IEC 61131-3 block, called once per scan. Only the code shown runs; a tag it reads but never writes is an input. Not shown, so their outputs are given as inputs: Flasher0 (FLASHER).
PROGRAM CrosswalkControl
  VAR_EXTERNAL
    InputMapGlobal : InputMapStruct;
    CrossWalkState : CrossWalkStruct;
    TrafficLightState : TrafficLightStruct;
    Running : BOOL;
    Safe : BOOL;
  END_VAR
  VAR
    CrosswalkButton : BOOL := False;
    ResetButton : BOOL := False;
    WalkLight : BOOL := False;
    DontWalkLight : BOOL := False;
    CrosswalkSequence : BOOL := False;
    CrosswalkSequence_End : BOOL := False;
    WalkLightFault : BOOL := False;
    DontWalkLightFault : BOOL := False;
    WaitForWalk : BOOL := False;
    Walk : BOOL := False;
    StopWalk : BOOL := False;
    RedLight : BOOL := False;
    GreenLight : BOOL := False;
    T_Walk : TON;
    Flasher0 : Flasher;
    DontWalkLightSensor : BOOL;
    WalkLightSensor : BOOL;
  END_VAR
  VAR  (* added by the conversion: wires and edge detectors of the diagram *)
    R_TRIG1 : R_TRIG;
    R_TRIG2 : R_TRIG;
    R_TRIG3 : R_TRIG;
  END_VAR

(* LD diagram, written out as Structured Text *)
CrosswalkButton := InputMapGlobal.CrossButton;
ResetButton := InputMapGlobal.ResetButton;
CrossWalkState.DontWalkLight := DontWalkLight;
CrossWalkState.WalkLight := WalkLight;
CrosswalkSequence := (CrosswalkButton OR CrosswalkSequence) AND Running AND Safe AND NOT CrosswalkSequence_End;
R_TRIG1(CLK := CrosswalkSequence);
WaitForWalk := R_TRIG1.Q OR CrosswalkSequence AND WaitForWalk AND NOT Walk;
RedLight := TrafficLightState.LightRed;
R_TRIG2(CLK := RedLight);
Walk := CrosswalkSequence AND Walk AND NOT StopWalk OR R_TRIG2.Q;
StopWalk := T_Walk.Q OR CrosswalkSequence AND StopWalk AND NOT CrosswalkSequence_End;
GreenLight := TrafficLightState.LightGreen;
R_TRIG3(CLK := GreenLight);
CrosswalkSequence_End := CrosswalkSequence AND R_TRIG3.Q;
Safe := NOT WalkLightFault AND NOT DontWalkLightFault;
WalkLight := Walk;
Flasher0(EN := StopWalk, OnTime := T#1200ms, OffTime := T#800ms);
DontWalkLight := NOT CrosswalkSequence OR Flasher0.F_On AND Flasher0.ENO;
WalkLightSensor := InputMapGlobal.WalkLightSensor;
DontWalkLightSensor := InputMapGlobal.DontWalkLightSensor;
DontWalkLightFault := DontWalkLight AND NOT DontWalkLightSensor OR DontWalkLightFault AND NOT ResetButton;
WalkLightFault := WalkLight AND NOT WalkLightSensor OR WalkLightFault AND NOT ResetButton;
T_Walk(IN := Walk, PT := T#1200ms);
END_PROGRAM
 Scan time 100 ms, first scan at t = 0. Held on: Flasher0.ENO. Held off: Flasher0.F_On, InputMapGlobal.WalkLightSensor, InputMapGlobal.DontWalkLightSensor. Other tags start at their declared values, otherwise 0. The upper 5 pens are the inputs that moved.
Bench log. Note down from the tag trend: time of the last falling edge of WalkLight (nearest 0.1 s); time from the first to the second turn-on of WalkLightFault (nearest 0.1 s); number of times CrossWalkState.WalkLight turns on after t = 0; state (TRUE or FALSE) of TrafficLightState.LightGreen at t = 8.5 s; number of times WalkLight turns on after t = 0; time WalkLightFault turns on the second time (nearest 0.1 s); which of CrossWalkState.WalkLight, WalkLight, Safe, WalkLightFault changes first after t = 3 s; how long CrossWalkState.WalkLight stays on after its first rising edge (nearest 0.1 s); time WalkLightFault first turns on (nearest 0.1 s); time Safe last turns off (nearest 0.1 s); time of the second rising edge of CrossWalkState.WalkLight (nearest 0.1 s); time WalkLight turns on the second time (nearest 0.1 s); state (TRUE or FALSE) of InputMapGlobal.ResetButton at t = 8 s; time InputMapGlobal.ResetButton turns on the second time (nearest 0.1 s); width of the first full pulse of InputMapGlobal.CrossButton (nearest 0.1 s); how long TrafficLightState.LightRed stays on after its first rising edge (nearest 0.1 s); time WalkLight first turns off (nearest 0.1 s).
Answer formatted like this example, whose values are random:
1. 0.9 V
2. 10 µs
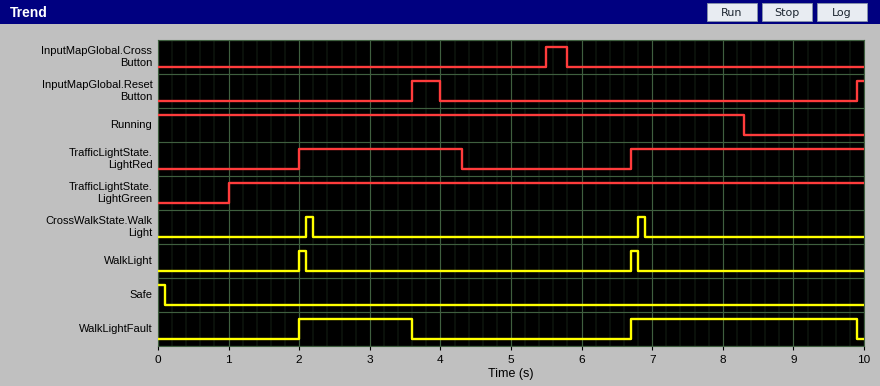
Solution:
1. 6.8 s
2. 4.7 s
3. 2
4. TRUE
5. 2
6. 6.7 s
7. WalkLightFault
8. 0.1 s
9. 2.0 s
10. 0.1 s
11. 6.8 s
12. 6.7 s
13. FALSE
14. 9.9 s
15. 0.3 s
16. 2.3 s
17. 2.1 s
